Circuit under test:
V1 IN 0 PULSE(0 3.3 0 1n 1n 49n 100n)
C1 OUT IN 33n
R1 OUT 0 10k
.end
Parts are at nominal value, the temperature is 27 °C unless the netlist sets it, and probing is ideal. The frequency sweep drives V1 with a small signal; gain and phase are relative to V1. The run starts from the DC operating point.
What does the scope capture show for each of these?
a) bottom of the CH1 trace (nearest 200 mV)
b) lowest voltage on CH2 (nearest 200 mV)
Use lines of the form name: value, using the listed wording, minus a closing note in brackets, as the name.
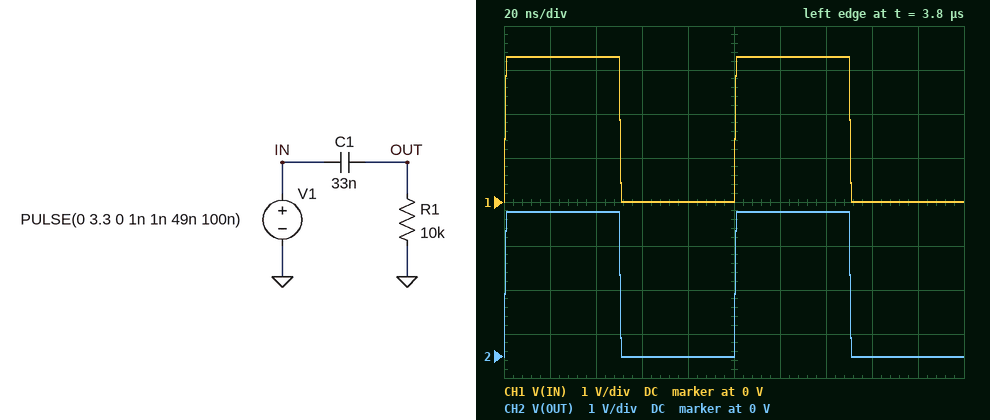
bottom of the CH1 trace: 0 V
lowest voltage on CH2: 0 V
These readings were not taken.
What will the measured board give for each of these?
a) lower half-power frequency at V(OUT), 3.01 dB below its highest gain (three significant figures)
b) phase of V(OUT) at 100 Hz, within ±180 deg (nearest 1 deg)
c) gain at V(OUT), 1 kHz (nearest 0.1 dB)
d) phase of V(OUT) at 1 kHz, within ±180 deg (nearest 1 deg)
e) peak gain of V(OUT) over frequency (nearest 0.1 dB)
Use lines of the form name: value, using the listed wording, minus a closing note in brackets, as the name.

lower half-power frequency at V(OUT), 3.01 dB below its highest gain: 482 Hz
phase of V(OUT) at 100 Hz, within ±180 deg: 78 deg
gain at V(OUT), 1 kHz: -0.9 dB
phase of V(OUT) at 1 kHz, within ±180 deg: 26 deg
peak gain of V(OUT) over frequency: 0 dB
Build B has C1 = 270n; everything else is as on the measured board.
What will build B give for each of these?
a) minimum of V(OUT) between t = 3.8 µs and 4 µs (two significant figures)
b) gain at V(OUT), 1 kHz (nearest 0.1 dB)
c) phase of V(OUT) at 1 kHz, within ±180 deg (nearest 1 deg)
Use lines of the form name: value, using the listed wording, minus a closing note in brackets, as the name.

minimum of V(OUT) between t = 3.8 µs and 4 µs: -2.4 mV
gain at V(OUT), 1 kHz: 0 dB
phase of V(OUT) at 1 kHz, within ±180 deg: 3 deg
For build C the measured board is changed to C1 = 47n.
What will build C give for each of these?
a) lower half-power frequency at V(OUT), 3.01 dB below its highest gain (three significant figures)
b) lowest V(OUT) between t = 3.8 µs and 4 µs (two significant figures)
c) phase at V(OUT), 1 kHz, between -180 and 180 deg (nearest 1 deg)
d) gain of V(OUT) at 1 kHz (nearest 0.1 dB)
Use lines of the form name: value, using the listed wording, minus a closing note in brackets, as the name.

lower half-power frequency at V(OUT), 3.01 dB below its highest gain: 339 Hz
lowest V(OUT) between t = 3.8 µs and 4 µs: -14 mV
phase at V(OUT), 1 kHz, between -180 and 180 deg: 19 deg
gain of V(OUT) at 1 kHz: -0.5 dB
